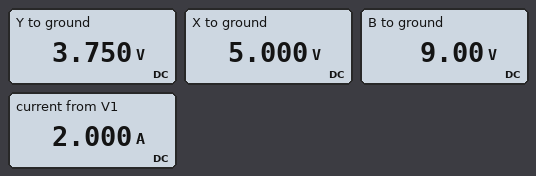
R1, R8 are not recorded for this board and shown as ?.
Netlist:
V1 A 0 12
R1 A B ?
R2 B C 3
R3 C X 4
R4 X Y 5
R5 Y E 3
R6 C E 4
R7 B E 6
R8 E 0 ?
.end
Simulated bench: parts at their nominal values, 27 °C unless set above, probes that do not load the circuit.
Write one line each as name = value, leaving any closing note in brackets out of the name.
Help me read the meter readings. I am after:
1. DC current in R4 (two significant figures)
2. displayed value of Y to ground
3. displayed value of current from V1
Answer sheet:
DC current in R4 = 250 mA
displayed value of Y to ground = 3.750 V
displayed value of current from V1 = 2.000 A
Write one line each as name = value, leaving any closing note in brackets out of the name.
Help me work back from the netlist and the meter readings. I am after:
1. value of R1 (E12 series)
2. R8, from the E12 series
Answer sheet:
value of R1 = 1.5 Ω
R8, from the E12 series = 1.5 Ω
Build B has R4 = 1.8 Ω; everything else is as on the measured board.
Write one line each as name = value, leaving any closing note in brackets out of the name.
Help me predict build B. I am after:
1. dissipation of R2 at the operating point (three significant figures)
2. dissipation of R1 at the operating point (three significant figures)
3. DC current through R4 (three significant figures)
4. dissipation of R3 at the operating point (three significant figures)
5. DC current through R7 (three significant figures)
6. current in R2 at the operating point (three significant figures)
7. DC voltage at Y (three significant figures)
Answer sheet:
dissipation of R2 at the operating point = 3.20 W
dissipation of R1 at the operating point = 6.13 W
DC current through R4 = 323 mA
dissipation of R3 at the operating point = 416 mW
DC current through R7 = 989 mA
current in R2 at the operating point = 1.03 A
DC voltage at Y = 4.00 V
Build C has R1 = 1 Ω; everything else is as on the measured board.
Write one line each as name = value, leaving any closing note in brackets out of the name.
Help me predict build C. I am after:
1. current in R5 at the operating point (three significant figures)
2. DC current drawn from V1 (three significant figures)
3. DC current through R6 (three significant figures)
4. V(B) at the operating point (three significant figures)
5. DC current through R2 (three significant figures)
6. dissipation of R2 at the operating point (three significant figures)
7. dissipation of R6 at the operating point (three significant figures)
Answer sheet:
current in R5 at the operating point = 273 mA
DC current drawn from V1 = 2.18 A
DC current through R6 = 818 mA
V(B) at the operating point = 9.82 V
DC current through R2 = 1.09 A
dissipation of R2 at the operating point = 3.57 W
dissipation of R6 at the operating point = 2.68 W
